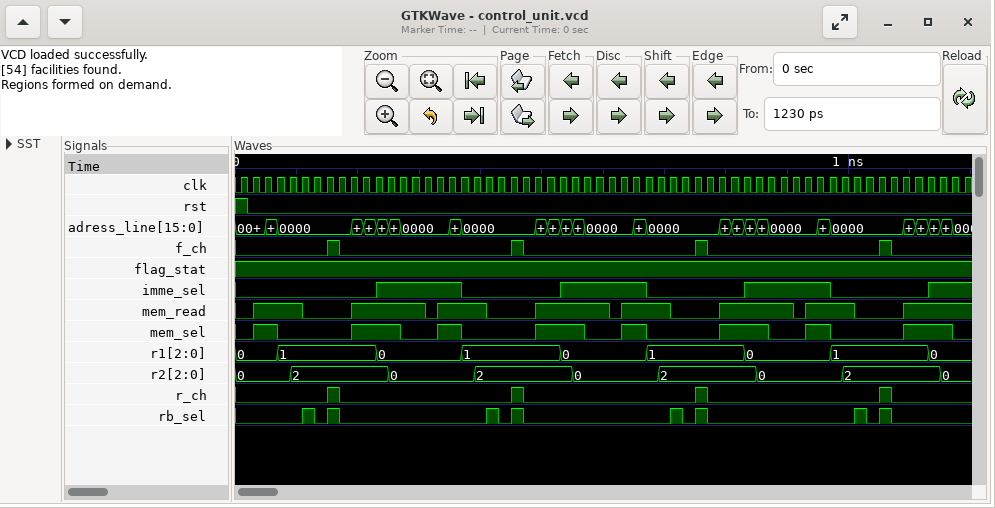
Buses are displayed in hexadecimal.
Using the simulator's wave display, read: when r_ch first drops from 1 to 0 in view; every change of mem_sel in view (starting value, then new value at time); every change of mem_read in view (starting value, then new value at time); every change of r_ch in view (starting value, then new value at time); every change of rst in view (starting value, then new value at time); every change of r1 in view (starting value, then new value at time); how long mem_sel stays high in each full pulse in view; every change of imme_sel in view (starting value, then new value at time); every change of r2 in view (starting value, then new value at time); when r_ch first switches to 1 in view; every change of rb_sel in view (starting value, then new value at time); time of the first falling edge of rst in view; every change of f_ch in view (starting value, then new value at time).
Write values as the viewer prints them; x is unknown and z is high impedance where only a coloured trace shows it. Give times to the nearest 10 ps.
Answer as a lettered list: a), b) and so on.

a) 170 ps
b) 0, 1 at 30 ps, 0 at 70 ps, 1 at 190 ps, 0 at 270 ps, 1 at 330 ps, 0 at 370 ps, 1 at 490 ps, 0 at 570 ps, 1 at 630 ps, 0 at 670 ps, 1 at 790 ps, 0 at 870 ps, 1 at 930 ps, 0 at 970 ps, 1 at 1090 ps, 0 at 1170 ps
c) 0, 1 at 30 ps, 0 at 110 ps, 1 at 190 ps, 0 at 310 ps, 1 at 330 ps, 0 at 410 ps, 1 at 490 ps, 0 at 610 ps, 1 at 630 ps, 0 at 710 ps, 1 at 790 ps, 0 at 910 ps, 1 at 930 ps, 0 at 1010 ps, 1 at 1090 ps
d) 0, 1 at 150 ps, 0 at 170 ps, 1 at 450 ps, 0 at 470 ps, 1 at 750 ps, 0 at 770 ps, 1 at 1050 ps, 0 at 1070 ps
e) 1, 0 at 20 ps
f) 0, 1 at 70 ps, 0 at 230 ps, 1 at 370 ps, 0 at 530 ps, 1 at 670 ps, 0 at 830 ps, 1 at 970 ps, 0 at 1130 ps
g) 40 ps, 80 ps, 40 ps, 80 ps, 40 ps, 80 ps, 40 ps, 80 ps
h) 0, 1 at 230 ps, 0 at 370 ps, 1 at 530 ps, 0 at 670 ps, 1 at 830 ps, 0 at 970 ps, 1 at 1130 ps
i) 0, 2 at 90 ps, 0 at 250 ps, 2 at 390 ps, 0 at 550 ps, 2 at 690 ps, 0 at 850 ps, 2 at 990 ps, 0 at 1150 ps
j) 150 ps
k) 0, 1 at 110 ps, 0 at 130 ps, 1 at 150 ps, 0 at 170 ps, 1 at 410 ps, 0 at 430 ps, 1 at 450 ps, 0 at 470 ps, 1 at 710 ps, 0 at 730 ps, 1 at 750 ps, 0 at 770 ps, 1 at 1010 ps, 0 at 1030 ps, 1 at 1050 ps, 0 at 1070 ps
l) 20 ps
m) 0, 1 at 150 ps, 0 at 170 ps, 1 at 450 ps, 0 at 470 ps, 1 at 750 ps, 0 at 770 ps, 1 at 1050 ps, 0 at 1070 ps
